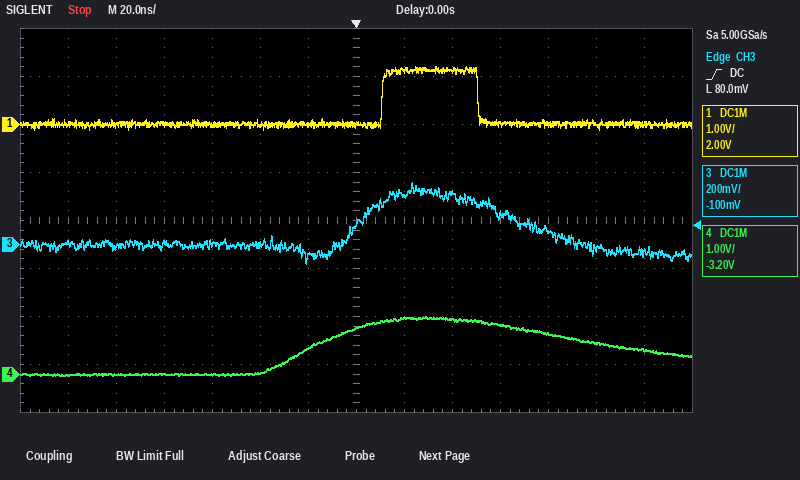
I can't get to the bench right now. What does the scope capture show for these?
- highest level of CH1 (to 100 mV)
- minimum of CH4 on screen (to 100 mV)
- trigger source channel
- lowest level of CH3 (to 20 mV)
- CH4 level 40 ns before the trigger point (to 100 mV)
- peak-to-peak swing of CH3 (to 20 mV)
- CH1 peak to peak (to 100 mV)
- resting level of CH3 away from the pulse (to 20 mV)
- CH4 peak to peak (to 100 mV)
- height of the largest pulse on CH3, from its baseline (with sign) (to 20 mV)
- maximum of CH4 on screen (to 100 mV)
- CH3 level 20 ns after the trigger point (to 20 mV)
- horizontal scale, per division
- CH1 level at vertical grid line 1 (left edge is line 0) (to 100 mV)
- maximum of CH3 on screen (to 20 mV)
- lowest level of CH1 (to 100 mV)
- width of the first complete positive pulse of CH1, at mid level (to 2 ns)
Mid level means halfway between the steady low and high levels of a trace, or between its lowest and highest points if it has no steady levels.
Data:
1.2 V
0.0 V
CH3
-80 mV
0.0 V
340 mV
1.3 V
0 mV
1.2 V
+260 mV
1.2 V
200 mV
20 ns
0.0 V
260 mV
-100 mV
40 ns
